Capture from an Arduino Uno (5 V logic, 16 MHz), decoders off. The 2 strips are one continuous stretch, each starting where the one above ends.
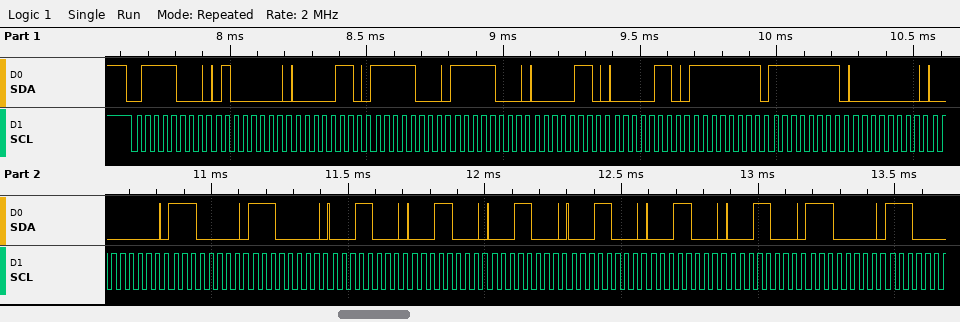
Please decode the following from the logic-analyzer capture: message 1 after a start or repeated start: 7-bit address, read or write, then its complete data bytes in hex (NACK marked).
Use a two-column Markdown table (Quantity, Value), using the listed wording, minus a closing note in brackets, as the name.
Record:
| Quantity | Value |
|---|---|
| message 1 after a start or repeated start: 7-bit address, read or write, then its complete data bytes in hex | 0x3C write: 40 06 F8 F8 06 06 FF FF 00 00 E0 E0 18 18 18 18 18 18 E0 |
